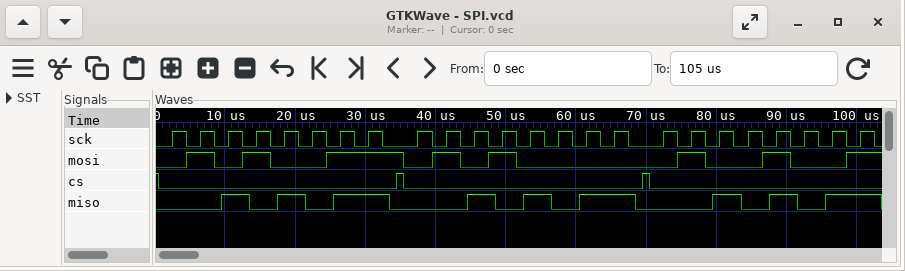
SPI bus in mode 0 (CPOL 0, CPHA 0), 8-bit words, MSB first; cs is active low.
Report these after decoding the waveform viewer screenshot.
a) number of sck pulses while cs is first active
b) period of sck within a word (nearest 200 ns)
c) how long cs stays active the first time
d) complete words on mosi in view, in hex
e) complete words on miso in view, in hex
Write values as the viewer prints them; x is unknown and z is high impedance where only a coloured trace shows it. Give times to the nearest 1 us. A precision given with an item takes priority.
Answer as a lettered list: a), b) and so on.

a) 8
b) 4000 ns
c) 34 us
d) 53, 50, 49
e) 2B, 2B, 2B
